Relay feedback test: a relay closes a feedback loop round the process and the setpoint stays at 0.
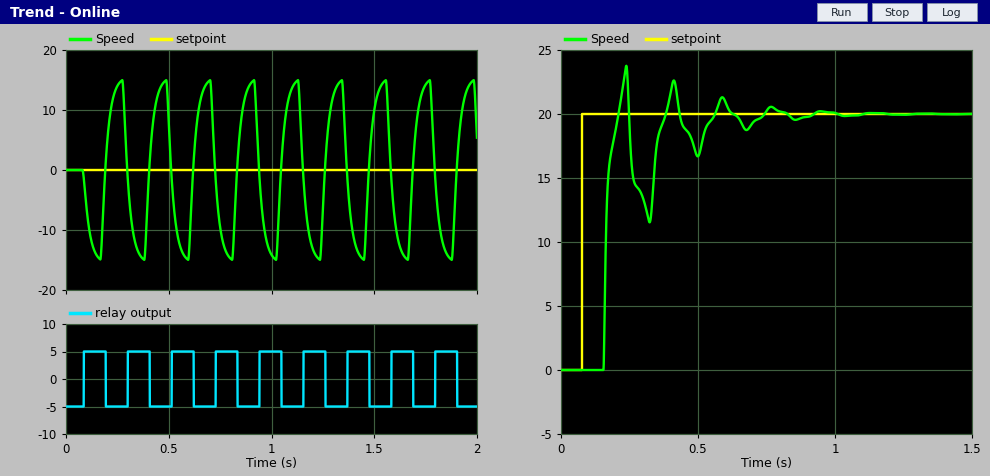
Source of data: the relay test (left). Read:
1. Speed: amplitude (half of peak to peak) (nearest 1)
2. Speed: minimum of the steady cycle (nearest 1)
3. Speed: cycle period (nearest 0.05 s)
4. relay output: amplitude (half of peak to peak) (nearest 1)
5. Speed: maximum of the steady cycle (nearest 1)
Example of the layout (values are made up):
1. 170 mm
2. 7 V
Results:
1. 15
2. -15
3. 0.20 s
4. 5
5. 15
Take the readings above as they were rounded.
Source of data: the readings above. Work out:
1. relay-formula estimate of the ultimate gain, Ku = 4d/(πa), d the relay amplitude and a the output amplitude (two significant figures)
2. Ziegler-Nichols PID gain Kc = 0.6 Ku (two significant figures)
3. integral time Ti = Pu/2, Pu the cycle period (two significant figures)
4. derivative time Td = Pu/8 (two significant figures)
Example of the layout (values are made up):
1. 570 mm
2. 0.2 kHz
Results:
1. 0.42
2. 0.25
3. 0.10 s
4. 0.025 s
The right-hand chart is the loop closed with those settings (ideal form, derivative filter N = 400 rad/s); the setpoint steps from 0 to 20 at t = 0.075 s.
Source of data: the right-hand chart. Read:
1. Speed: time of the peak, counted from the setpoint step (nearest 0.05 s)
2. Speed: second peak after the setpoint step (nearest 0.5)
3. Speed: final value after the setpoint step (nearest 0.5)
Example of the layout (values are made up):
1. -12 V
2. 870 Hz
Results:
1. 0.15 s
2. 22.5
3. 20.0
